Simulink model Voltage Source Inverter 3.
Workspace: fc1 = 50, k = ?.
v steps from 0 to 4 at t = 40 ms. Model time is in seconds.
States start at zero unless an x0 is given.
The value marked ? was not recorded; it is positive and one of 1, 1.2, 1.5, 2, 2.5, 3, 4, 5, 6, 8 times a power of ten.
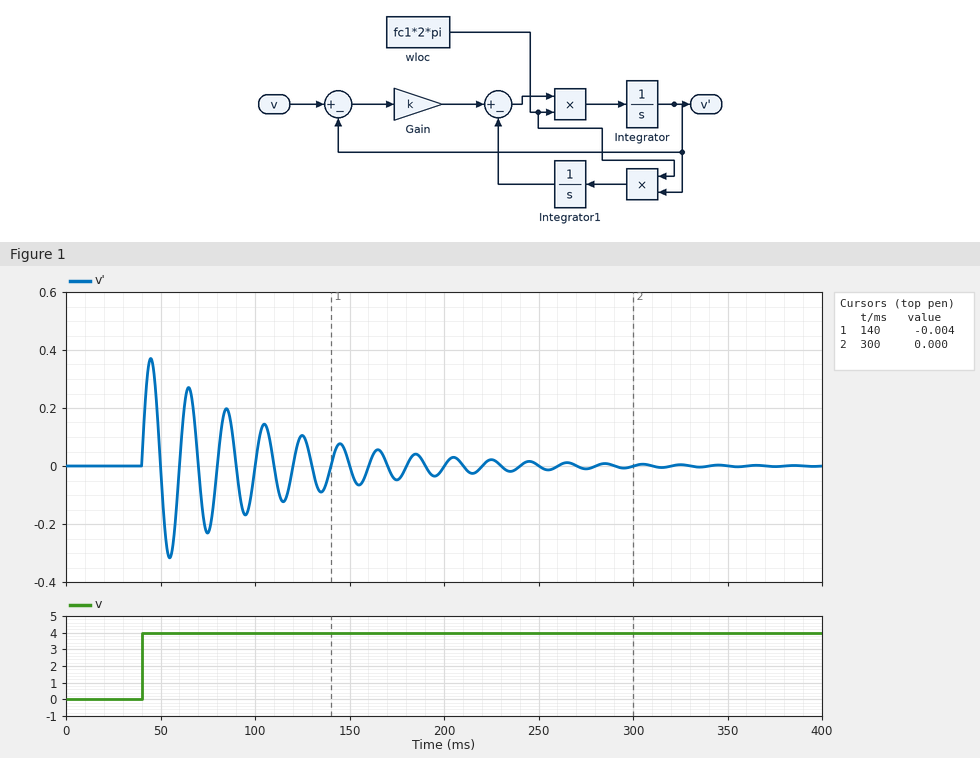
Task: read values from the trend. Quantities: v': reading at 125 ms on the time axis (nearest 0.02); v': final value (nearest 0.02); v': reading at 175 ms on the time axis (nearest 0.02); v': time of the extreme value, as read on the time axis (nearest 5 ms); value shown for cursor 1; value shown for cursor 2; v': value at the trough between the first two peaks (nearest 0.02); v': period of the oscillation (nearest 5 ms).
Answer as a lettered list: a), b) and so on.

a) 0.10
b) 0.00
c) -0.04
d) 45 ms
e) -0.004
f) 0.000
g) -0.32
h) 20 ms
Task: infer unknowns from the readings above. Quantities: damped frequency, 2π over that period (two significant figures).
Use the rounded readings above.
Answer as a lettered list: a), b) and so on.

a) 0.31 rad/ms
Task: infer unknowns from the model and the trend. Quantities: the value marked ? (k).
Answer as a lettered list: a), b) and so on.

a) 0.1
